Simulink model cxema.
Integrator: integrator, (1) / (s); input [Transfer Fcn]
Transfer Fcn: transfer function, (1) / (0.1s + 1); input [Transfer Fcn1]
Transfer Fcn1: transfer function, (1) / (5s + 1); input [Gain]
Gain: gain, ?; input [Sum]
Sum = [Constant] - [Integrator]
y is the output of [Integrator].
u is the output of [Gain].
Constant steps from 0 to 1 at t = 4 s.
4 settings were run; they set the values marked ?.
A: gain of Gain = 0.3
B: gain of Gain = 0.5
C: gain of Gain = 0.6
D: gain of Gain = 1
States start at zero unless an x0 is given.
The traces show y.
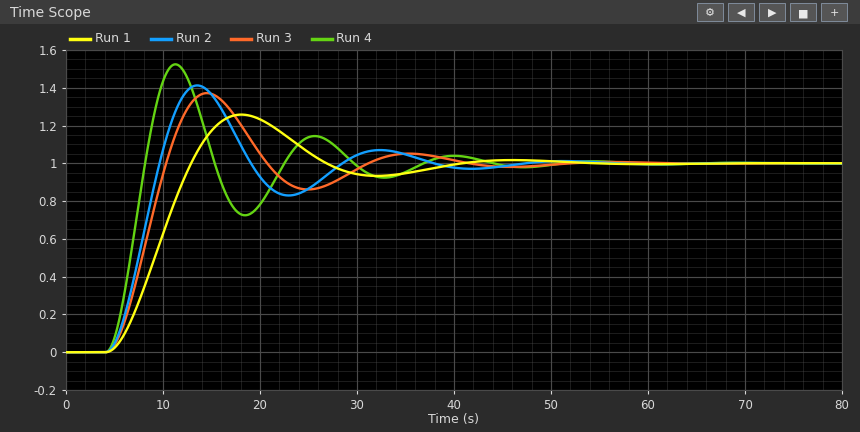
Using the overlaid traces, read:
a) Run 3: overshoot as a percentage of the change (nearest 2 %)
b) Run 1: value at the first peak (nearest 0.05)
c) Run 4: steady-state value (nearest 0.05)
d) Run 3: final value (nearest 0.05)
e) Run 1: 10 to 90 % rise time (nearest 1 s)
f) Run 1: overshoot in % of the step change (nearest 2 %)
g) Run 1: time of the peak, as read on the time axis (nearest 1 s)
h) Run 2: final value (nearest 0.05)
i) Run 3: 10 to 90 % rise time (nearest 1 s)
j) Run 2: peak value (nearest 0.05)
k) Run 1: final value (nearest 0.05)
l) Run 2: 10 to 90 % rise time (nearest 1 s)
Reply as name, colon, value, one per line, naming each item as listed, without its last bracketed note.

Run 3: overshoot as a percentage of the change: 38 %
Run 1: value at the first peak: 1.25
Run 4: steady-state value: 1.00
Run 3: final value: 1.00
Run 1: 10 to 90 % rise time: 6 s
Run 1: overshoot in % of the step change: 26 %
Run 1: time of the peak, as read on the time axis: 18 s
Run 2: final value: 1.00
Run 3: 10 to 90 % rise time: 4 s
Run 2: peak value: 1.40
Run 1: final value: 1.00
Run 2: 10 to 90 % rise time: 4 s
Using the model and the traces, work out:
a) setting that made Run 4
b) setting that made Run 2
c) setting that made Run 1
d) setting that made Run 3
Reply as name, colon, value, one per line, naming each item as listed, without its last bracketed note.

setting that made Run 4: D
setting that made Run 2: C
setting that made Run 1: A
setting that made Run 3: B
